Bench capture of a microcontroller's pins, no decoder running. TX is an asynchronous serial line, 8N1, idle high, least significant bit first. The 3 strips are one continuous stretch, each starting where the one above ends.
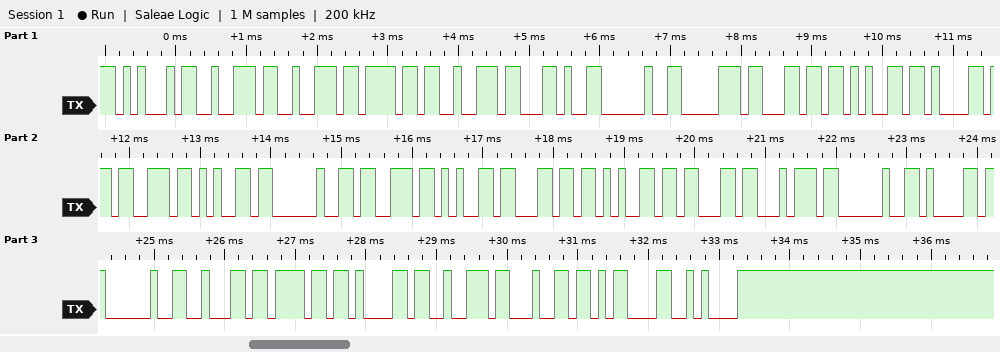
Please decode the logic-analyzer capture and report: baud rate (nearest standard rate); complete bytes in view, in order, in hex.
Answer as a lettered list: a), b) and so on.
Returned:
a) 9600 baud
b) 45 72 72 6F 72 2C 20 70 6C 65 61 73 65 20 73 65 6C 65 63 74 20 61 20 62 6F 61 72 64 0D 0A
